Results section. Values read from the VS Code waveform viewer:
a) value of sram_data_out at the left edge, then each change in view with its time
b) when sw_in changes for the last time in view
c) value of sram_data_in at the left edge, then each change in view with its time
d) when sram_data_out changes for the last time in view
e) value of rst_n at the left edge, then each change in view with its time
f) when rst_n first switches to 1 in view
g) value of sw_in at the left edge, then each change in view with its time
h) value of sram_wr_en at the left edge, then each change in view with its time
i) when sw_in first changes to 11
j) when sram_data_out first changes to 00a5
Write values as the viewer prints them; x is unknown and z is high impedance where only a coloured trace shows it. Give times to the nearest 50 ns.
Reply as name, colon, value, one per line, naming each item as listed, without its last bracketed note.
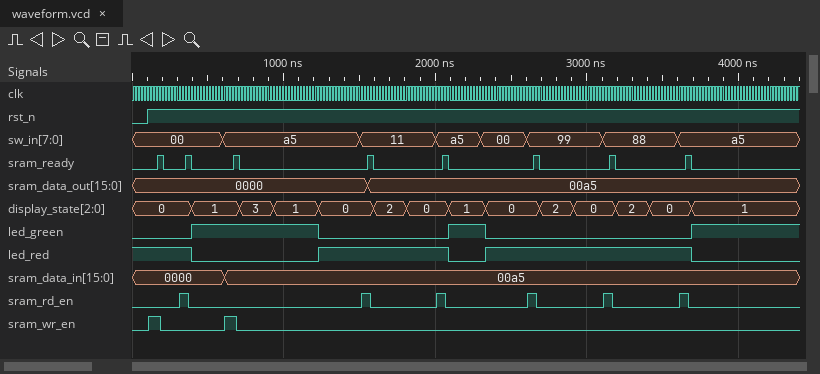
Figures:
value of sram_data_out at the left edge, then each change in view with its time: 0000, 00a5 at 1550 ns
when sw_in changes for the last time in view: 3600 ns
value of sram_data_in at the left edge, then each change in view with its time: 0000, 00a5 at 600 ns
when sram_data_out changes for the last time in view: 1550 ns
value of rst_n at the left edge, then each change in view with its time: 0, 1 at 100 ns
when rst_n first switches to 1 in view: 100 ns
value of sw_in at the left edge, then each change in view with its time: 00, a5 at 600 ns, 11 at 1500 ns, a5 at 2000 ns, 00 at 2300 ns, 99 at 2600 ns, 88 at 3100 ns, a5 at 3600 ns
value of sram_wr_en at the left edge, then each change in view with its time: 0, 1 at 100 ns, 0 at 200 ns, 1 at 600 ns, 0 at 700 ns
when sw_in first changes to 11: 1500 ns
when sram_data_out first changes to 00a5: 1550 ns
